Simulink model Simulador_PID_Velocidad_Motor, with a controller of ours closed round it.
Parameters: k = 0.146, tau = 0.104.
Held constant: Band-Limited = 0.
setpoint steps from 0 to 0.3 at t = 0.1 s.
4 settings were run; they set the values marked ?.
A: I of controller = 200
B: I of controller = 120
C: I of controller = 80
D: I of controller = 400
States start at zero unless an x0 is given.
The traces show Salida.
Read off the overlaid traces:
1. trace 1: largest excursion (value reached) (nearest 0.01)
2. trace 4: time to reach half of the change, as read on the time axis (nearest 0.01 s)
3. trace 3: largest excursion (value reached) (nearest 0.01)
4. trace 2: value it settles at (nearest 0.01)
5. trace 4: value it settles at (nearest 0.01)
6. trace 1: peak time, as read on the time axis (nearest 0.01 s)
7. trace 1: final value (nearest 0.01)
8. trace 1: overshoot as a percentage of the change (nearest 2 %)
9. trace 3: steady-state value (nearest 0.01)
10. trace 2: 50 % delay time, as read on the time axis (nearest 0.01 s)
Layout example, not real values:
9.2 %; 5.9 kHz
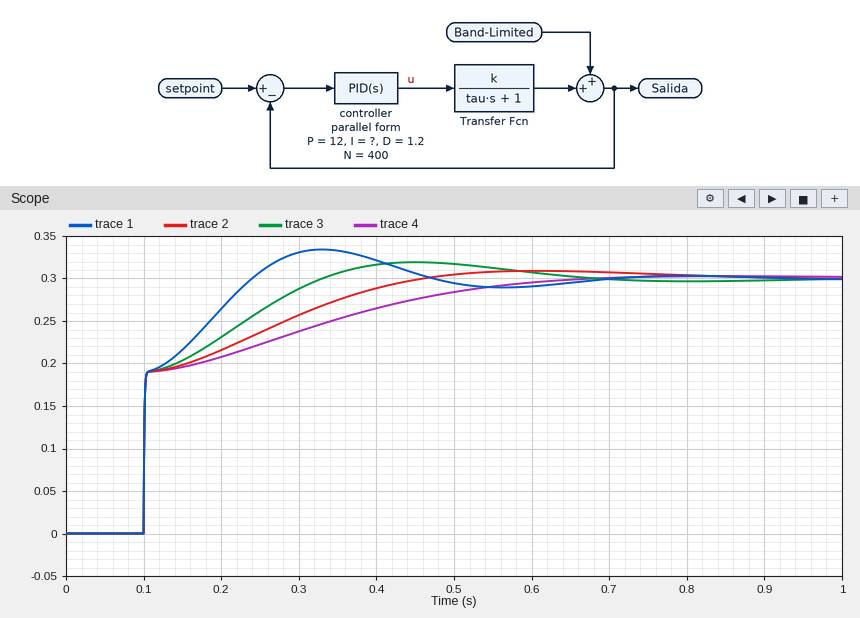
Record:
0.33; 0.10 s; 0.32; 0.30; 0.30; 0.33 s; 0.30; 12 %; 0.30; 0.10 s
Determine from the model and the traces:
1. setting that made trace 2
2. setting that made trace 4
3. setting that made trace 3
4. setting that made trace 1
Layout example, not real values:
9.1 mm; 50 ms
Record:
B; C; A; D
